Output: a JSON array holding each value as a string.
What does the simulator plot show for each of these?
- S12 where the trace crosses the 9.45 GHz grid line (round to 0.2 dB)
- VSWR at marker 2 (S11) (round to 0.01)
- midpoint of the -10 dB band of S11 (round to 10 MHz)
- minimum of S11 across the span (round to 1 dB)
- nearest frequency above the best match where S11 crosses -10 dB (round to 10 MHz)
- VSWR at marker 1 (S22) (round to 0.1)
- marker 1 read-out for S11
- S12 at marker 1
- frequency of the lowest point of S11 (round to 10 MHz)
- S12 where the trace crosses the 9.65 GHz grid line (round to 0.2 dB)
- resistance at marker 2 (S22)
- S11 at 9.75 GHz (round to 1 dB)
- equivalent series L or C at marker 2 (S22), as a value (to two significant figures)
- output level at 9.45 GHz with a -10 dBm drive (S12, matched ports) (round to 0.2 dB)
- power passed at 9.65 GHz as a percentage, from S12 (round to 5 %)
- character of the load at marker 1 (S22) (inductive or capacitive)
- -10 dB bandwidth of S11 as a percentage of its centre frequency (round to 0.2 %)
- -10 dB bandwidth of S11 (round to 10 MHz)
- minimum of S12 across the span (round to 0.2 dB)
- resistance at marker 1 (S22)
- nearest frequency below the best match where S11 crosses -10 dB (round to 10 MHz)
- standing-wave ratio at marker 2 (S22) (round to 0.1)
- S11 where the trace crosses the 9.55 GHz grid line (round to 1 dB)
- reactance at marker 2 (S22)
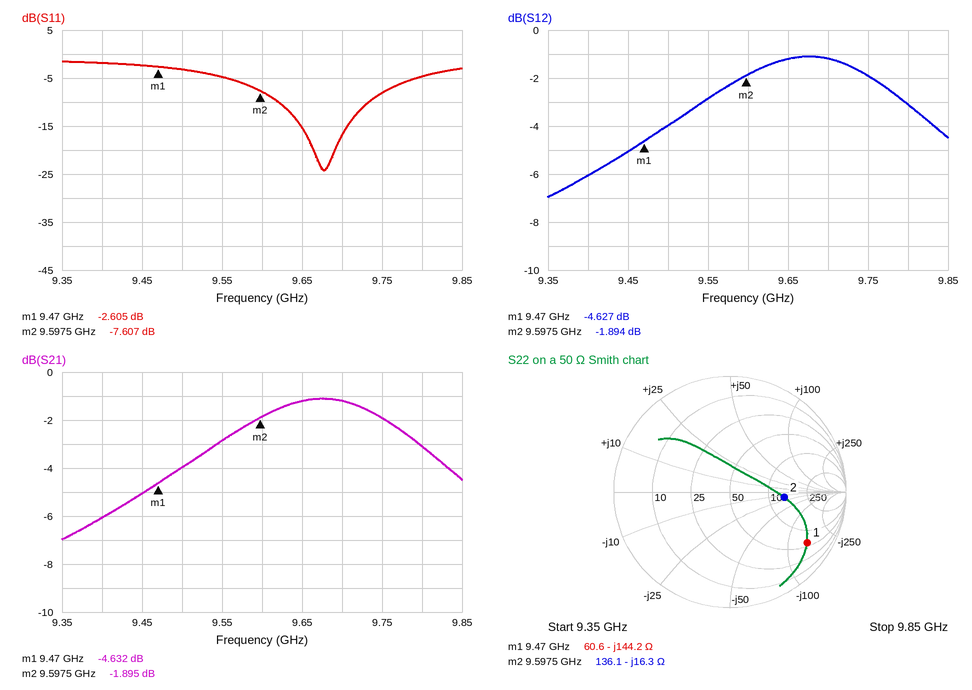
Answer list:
["-5.0 dB", "2.43", "9.68 GHz", "-24 dB", "9.73 GHz", "8.8", "-2.605 dB", "-4.627 dB", "9.68 GHz", "-1.2 dB", "136.1 Ω", "-8 dB", "1.0 pF", "-15.0 dBm", "75 %", "capacitive", "1.2 %", "110 MHz", "-7.0 dB", "60.6 Ω", "9.62 GHz", "2.8", "-5 dB", "-16.3 Ω"]
